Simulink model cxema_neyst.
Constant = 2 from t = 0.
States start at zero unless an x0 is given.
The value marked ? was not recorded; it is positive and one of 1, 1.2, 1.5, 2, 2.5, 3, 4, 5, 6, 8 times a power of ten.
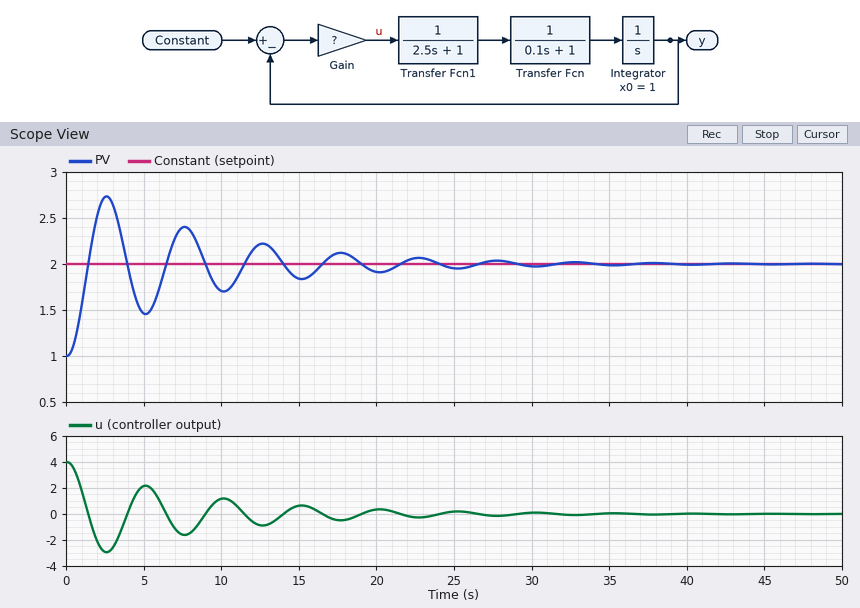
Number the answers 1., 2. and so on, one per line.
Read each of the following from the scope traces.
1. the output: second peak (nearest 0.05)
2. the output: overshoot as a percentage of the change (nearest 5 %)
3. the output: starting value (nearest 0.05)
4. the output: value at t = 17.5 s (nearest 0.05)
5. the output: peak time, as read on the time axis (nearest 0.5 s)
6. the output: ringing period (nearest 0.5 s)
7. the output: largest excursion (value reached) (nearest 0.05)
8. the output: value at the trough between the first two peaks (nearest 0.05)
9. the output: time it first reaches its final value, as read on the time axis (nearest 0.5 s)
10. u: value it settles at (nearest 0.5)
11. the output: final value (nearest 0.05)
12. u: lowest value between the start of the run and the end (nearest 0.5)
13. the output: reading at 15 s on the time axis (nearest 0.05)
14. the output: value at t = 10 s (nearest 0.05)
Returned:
1. 2.40
2. 75 %
3. 1.00
4. 2.10
5. 2.5 s
6. 5.0 s
7. 2.75
8. 1.45
9. 1.5 s
10. 0.0
11. 2.00
12. -3.0
13. 1.85
14. 1.70
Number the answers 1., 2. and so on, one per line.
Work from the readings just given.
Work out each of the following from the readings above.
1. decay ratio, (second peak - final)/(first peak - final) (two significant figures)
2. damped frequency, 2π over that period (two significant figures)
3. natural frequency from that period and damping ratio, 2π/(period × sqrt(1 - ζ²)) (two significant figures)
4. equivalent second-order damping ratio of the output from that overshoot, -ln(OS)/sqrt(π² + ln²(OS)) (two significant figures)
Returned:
1. 0.53
2. 1.3 rad/s
3. 1.3 rad/s
4. 0.091
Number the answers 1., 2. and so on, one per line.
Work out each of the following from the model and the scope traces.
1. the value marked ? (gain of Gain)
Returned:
1. 4
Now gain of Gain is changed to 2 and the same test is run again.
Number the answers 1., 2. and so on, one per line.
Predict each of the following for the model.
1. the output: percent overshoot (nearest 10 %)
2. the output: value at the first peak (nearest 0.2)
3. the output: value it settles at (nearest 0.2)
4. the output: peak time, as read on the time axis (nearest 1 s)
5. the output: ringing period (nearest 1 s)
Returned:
1. 60 %
2. 2.6
3. 2.0
4. 4 s
5. 7 s
